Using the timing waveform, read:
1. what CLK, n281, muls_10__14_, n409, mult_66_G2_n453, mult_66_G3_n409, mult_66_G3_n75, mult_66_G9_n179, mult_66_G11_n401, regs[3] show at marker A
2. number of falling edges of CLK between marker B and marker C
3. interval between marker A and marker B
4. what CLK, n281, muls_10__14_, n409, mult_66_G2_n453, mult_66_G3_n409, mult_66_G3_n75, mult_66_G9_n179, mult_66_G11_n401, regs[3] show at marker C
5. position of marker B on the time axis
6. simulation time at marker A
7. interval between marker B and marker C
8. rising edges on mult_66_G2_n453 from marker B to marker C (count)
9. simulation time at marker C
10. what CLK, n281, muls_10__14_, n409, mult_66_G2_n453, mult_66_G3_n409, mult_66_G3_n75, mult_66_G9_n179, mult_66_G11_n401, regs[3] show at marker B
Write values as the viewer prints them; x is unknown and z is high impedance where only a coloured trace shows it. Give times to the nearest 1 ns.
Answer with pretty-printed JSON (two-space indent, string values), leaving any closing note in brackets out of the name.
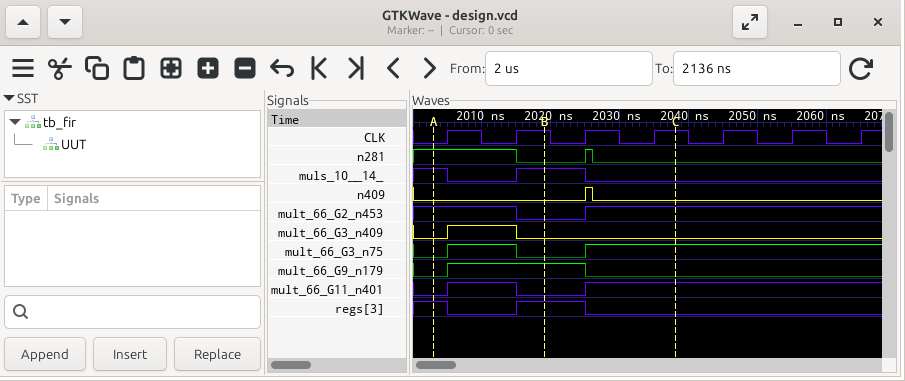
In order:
{
  "what CLK, n281, muls_10__14_, n409, mult_66_G2_n453, mult_66_G3_n409, mult_66_G3_n75, mult_66_G9_n179, mult_66_G11_n401, regs[3] show at marker A": "CLK=0, n281=1, muls_10__14_=1, n409=0, mult_66_G2_n453=1, mult_66_G3_n409=0, mult_66_G3_n75=0, mult_66_G9_n179=0, mult_66_G11_n401=0, regs[3]=1",
  "number of falling edges of CLK between marker B and marker C": "2",
  "interval between marker A and marker B": "16 ns",
  "what CLK, n281, muls_10__14_, n409, mult_66_G2_n453, mult_66_G3_n409, mult_66_G3_n75, mult_66_G9_n179, mult_66_G11_n401, regs[3] show at marker C": "CLK=1, n281=0, muls_10__14_=0, n409=0, mult_66_G2_n453=1, mult_66_G3_n409=0, mult_66_G3_n75=1, mult_66_G9_n179=0, mult_66_G11_n401=1, regs[3]=0",
  "position of marker B on the time axis": "2019 ns",
  "simulation time at marker A": "2003 ns",
  "interval between marker B and marker C": "19 ns",
  "rising edges on mult_66_G2_n453 from marker B to marker C": "1",
  "simulation time at marker C": "2038 ns",
  "what CLK, n281, muls_10__14_, n409, mult_66_G2_n453, mult_66_G3_n409, mult_66_G3_n75, mult_66_G9_n179, mult_66_G11_n401, regs[3] show at marker B": "CLK=1, n281=0, muls_10__14_=1, n409=0, mult_66_G2_n453=0, mult_66_G3_n409=0, mult_66_G3_n75=0, mult_66_G9_n179=1, mult_66_G11_n401=0, regs[3]=1"
}
